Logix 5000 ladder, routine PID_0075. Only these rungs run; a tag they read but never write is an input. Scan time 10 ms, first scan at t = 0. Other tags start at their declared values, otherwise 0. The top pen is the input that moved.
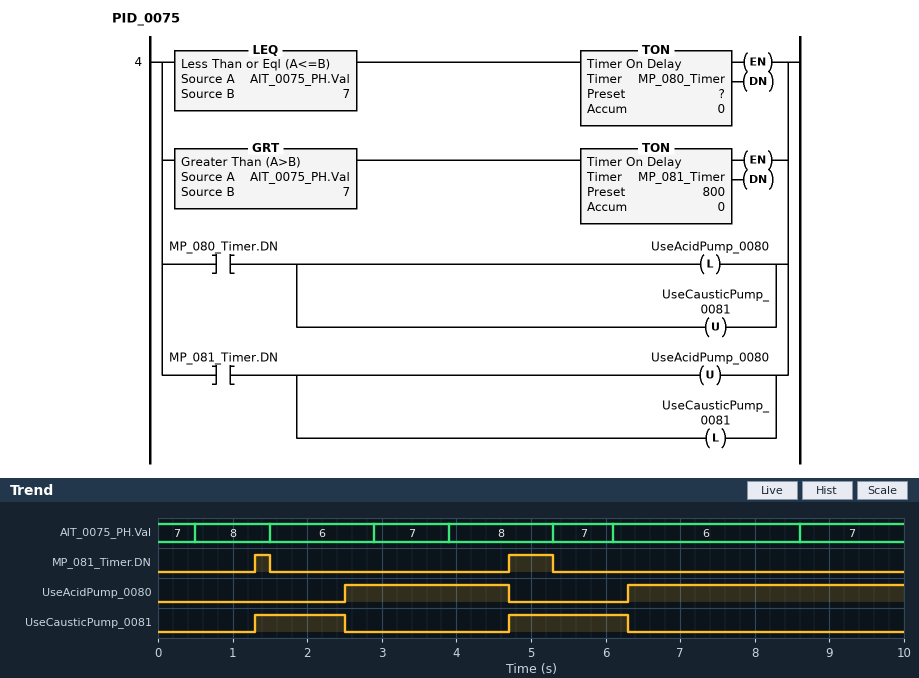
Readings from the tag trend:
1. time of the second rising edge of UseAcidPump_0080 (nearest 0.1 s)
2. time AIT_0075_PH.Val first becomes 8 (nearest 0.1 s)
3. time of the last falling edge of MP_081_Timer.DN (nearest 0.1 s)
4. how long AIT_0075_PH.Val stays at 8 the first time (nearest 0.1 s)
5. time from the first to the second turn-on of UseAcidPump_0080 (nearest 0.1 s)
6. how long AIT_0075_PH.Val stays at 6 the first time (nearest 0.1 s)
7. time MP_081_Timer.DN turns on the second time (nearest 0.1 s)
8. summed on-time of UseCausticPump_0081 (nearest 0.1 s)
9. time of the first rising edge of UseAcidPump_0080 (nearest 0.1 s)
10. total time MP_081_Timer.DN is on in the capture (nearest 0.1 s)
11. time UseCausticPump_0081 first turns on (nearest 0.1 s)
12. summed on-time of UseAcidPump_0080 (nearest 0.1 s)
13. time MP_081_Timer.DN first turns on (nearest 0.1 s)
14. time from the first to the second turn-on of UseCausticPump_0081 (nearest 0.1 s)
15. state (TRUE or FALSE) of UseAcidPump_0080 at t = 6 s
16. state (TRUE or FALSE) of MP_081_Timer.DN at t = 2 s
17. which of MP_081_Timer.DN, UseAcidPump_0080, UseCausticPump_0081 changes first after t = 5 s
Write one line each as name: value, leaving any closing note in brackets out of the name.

time of the second rising edge of UseAcidPump_0080: 6.3 s
time AIT_0075_PH.Val first becomes 8: 0.5 s
time of the last falling edge of MP_081_Timer.DN: 5.3 s
how long AIT_0075_PH.Val stays at 8 the first time: 1.0 s
time from the first to the second turn-on of UseAcidPump_0080: 3.8 s
how long AIT_0075_PH.Val stays at 6 the first time: 1.4 s
time MP_081_Timer.DN turns on the second time: 4.7 s
summed on-time of UseCausticPump_0081: 2.8 s
time of the first rising edge of UseAcidPump_0080: 2.5 s
total time MP_081_Timer.DN is on in the capture: 0.8 s
time UseCausticPump_0081 first turns on: 1.3 s
summed on-time of UseAcidPump_0080: 5.9 s
time MP_081_Timer.DN first turns on: 1.3 s
time from the first to the second turn-on of UseCausticPump_0081: 3.4 s
state (TRUE or FALSE) of UseAcidPump_0080 at t = 6 s: FALSE
state (TRUE or FALSE) of MP_081_Timer.DN at t = 2 s: FALSE
which of MP_081_Timer.DN, UseAcidPump_0080, UseCausticPump_0081 changes first after t = 5 s: MP_081_Timer.DN
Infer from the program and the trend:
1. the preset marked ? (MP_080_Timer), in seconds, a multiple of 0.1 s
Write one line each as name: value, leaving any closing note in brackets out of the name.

the preset marked ? (MP_080_Timer), in seconds, a multiple of 0.1 s: 1.0 s
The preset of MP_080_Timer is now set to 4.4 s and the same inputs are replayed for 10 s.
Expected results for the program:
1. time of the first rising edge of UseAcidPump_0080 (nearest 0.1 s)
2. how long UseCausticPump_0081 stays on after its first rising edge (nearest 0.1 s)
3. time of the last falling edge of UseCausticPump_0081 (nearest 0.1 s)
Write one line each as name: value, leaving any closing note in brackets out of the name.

time of the first rising edge of UseAcidPump_0080: 9.7 s
how long UseCausticPump_0081 stays on after its first rising edge: 8.4 s
time of the last falling edge of UseCausticPump_0081: 9.7 s
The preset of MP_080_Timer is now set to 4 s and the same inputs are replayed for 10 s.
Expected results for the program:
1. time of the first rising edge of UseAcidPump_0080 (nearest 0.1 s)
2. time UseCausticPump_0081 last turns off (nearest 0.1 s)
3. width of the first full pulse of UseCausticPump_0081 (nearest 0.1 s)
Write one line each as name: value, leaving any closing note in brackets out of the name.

time of the first rising edge of UseAcidPump_0080: 9.3 s
time UseCausticPump_0081 last turns off: 9.3 s
width of the first full pulse of UseCausticPump_0081: 8.0 s
